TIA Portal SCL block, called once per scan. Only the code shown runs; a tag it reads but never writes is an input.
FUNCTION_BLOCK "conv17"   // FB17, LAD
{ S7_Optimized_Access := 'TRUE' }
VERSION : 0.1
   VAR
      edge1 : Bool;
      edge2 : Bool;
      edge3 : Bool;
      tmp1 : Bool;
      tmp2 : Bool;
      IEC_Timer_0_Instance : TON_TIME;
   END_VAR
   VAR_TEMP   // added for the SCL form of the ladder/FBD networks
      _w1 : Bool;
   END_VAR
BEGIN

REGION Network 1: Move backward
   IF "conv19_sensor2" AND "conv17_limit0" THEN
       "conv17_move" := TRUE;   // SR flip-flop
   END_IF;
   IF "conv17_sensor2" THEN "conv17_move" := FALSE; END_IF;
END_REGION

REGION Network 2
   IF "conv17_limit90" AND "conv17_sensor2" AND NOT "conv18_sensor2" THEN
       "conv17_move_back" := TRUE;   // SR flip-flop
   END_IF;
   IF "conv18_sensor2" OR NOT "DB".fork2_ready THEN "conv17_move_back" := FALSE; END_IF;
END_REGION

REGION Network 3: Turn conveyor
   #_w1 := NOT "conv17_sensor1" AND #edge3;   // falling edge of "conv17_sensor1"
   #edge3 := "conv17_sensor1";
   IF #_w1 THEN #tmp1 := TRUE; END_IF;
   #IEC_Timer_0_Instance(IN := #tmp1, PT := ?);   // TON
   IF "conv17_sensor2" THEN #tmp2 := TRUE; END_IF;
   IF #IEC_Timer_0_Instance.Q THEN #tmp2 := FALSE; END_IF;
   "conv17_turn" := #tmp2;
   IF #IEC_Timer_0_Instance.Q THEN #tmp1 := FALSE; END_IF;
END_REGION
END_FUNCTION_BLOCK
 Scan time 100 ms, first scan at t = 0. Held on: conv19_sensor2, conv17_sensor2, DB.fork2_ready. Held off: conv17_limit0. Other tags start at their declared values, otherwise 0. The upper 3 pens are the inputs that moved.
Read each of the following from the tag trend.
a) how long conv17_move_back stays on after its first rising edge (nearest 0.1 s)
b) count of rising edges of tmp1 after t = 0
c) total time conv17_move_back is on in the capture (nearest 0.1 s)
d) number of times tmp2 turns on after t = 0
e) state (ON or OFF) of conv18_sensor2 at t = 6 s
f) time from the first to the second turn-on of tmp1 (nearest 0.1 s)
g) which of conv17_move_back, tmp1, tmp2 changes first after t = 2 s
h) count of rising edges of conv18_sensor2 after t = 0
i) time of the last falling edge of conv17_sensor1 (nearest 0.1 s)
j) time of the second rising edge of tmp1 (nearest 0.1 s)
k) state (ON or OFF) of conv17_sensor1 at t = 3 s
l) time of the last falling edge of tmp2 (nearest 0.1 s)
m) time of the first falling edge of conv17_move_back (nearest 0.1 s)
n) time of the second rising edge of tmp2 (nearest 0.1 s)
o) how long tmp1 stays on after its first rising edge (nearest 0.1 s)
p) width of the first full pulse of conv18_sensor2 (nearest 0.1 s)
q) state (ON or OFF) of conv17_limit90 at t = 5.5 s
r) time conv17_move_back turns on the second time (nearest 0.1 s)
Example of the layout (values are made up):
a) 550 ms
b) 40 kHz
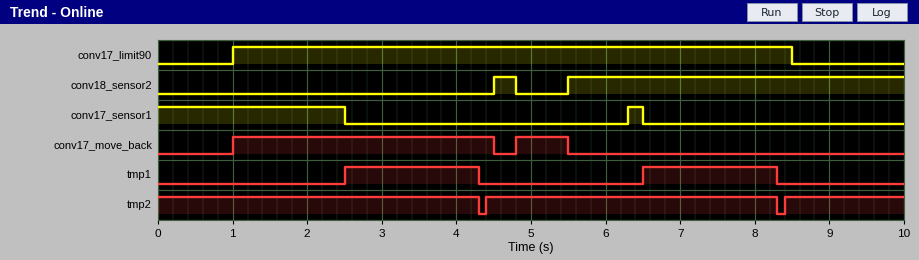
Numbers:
a) 3.5 s
b) 2
c) 4.2 s
d) 2
e) ON
f) 4.0 s
g) tmp1
h) 2
i) 6.5 s
j) 6.5 s
k) OFF
l) 8.3 s
m) 4.5 s
n) 8.4 s
o) 1.8 s
p) 0.3 s
q) ON
r) 4.8 s
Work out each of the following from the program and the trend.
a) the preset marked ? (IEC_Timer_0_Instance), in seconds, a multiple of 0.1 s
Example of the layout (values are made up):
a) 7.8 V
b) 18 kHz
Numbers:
a) 1.8 s
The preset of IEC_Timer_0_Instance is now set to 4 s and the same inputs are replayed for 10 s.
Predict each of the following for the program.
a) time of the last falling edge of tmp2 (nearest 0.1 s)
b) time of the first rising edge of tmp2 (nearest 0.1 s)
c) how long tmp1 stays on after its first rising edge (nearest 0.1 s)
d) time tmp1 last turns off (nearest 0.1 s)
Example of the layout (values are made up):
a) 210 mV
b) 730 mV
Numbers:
a) 6.5 s
b) 6.6 s
c) 4.0 s
d) 6.5 s
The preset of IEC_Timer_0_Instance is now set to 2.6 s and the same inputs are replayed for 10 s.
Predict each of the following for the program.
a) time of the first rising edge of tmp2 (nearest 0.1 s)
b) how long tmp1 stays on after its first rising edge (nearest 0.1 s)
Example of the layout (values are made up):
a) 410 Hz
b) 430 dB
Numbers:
a) 5.2 s
b) 2.6 s
